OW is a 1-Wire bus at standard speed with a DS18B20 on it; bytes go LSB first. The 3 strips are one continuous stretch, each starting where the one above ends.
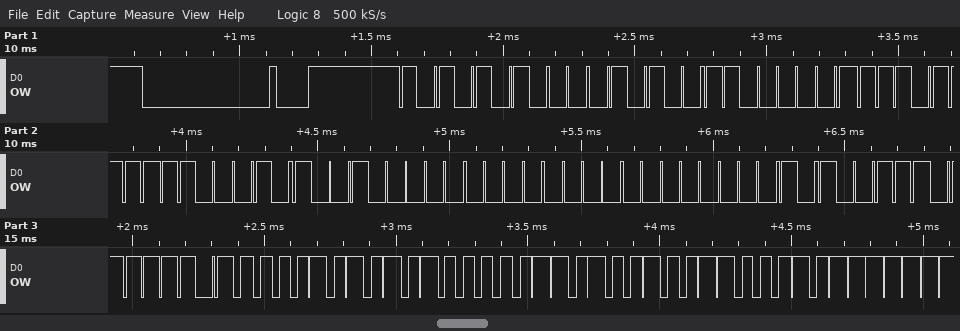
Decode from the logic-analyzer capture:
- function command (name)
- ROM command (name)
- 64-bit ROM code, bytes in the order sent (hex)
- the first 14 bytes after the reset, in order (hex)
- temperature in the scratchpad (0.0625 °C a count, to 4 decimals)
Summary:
Read Scratchpad
Match ROM
28 83 F7 A3 04 00 00 E5
55 28 83 F7 A3 04 00 00 E5 BE 50 05 4B 46
85.0000 °C
